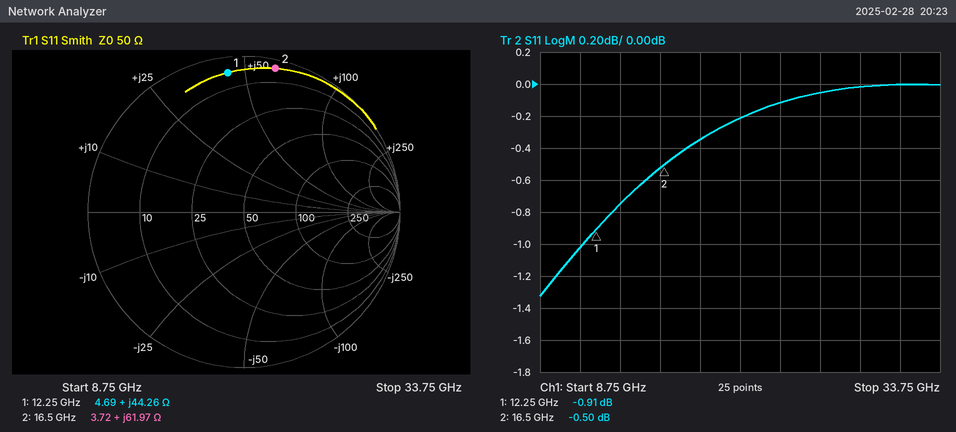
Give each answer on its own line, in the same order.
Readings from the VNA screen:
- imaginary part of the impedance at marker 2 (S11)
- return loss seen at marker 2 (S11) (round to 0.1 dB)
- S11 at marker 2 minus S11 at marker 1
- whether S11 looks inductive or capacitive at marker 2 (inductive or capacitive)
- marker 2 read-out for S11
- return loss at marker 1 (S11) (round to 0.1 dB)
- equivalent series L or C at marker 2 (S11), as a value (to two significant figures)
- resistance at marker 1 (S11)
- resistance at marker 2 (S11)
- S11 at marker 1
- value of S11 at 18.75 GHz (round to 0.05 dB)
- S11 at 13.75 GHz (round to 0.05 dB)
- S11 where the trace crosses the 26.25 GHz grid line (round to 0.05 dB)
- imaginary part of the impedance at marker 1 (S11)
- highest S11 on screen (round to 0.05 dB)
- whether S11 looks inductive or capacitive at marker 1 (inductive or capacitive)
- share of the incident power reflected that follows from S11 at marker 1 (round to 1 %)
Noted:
+61.97 Ω
0.5 dB
0.41 dB
inductive
-0.50 dB
0.9 dB
600 pH
4.69 Ω
3.72 Ω
-0.91 dB
-0.35 dB
-0.75 dB
-0.05 dB
+44.26 Ω
0.00 dB
inductive
81 %
